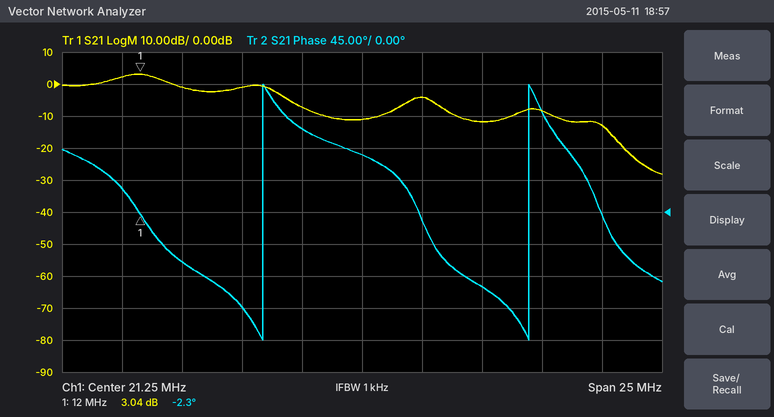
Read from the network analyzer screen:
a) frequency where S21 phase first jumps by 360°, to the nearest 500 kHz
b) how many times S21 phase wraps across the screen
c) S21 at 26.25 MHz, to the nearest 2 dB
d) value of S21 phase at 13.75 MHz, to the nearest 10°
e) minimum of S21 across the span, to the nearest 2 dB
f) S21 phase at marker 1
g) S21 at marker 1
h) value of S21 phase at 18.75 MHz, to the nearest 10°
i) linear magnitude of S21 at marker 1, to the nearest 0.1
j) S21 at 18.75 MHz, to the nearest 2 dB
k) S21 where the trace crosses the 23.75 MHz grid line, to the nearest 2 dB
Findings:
17.0 MHz
2
-12 dB
-70°
-28 dB
-2.3°
3.04 dB
120°
1.4
-8 dB
-4 dB
